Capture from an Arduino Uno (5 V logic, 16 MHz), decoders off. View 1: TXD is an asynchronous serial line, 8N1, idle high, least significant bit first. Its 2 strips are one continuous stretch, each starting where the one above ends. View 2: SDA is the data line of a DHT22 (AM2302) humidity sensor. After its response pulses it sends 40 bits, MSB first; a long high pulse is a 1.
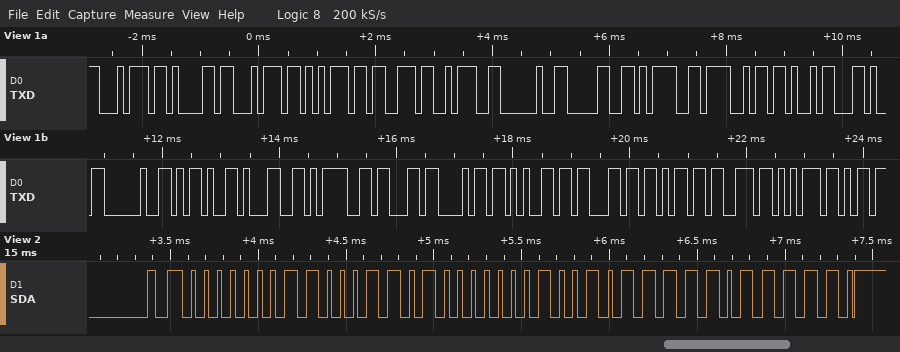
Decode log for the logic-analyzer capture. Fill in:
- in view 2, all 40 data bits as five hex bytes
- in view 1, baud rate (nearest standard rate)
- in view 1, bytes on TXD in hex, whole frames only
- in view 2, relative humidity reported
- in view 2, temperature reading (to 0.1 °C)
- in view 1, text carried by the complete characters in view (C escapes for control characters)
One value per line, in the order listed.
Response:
01 8D 01 2F BE
9600 baud
74 61 74 75 73 3A 20 30 3D 4F 4B 2C 20 2D 31 3D 63 68 65 63 6B 73 75
39.7 %
30.3 °C
"tatus: 0=OK, -1=checksu"
